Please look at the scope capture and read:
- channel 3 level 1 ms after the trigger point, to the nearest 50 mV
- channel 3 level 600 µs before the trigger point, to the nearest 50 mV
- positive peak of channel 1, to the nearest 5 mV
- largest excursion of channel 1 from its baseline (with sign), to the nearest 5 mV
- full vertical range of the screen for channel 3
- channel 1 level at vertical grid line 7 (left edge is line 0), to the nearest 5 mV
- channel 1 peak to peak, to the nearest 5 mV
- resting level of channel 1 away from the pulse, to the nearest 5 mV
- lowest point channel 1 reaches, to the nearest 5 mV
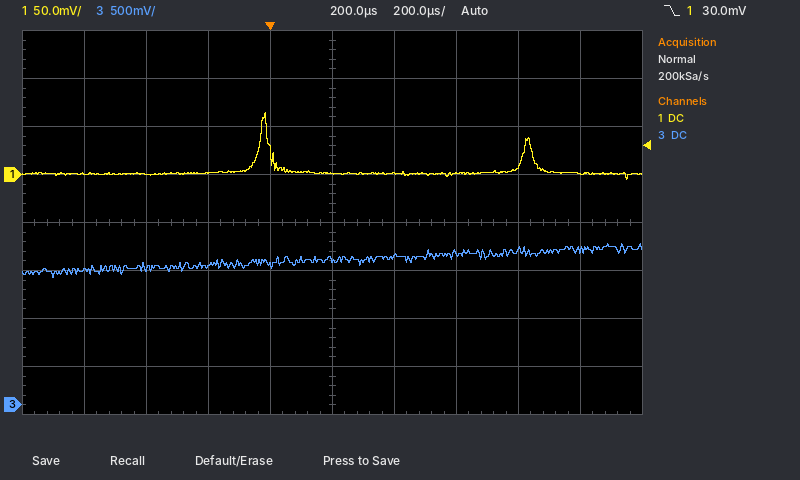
1.60 V
1.40 V
65 mV
+65 mV
4 V
0 mV
70 mV
0 mV
-5 mV
